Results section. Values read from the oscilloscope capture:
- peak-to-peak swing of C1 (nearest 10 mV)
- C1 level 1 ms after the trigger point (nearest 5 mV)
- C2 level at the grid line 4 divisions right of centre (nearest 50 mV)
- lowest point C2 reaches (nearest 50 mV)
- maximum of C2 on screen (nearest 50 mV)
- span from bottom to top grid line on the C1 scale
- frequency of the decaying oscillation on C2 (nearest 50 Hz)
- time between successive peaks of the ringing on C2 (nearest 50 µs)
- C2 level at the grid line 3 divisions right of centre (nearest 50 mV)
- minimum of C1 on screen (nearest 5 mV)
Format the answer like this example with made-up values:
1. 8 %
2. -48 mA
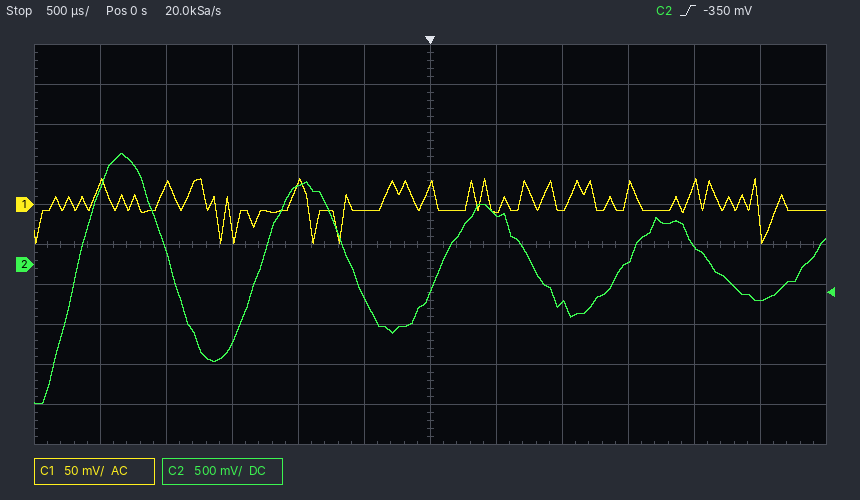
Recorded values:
1. 80 mV
2. -5 mV
3. 250 mV
4. -1.75 V
5. 1.40 V
6. 500 mV
7. 750 Hz
8. 1.35 ms
9. 50 mV
10. -50 mV
